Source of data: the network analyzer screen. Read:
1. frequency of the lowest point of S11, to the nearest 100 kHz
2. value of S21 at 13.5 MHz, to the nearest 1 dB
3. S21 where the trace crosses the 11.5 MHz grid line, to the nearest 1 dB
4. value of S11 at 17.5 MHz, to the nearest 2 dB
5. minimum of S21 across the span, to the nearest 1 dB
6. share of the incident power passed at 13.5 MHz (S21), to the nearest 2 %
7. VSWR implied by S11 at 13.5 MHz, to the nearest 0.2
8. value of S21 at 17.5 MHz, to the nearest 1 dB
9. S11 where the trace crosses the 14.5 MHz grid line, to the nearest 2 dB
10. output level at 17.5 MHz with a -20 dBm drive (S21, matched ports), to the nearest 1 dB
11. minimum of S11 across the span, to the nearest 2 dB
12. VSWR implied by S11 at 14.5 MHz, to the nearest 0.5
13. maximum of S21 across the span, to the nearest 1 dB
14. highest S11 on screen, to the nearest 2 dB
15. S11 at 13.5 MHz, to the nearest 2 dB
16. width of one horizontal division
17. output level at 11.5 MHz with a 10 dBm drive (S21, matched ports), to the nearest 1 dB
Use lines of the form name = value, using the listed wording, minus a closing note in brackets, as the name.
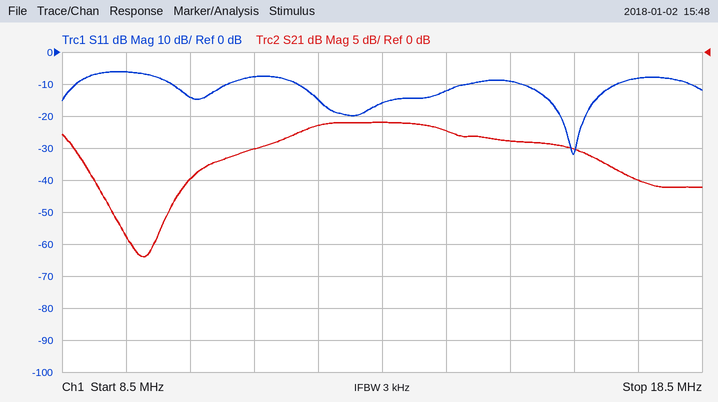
frequency of the lowest point of S11, to the nearest 100 kHz = 16.5 MHz
value of S21 at 13.5 MHz, to the nearest 1 dB = -11 dB
S21 where the trace crosses the 11.5 MHz grid line, to the nearest 1 dB = -15 dB
value of S11 at 17.5 MHz, to the nearest 2 dB = -8 dB
minimum of S21 across the span, to the nearest 1 dB = -32 dB
share of the incident power passed at 13.5 MHz (S21), to the nearest 2 % = 8 %
VSWR implied by S11 at 13.5 MHz, to the nearest 0.2 = 1.4
value of S21 at 17.5 MHz, to the nearest 1 dB = -20 dB
S11 where the trace crosses the 14.5 MHz grid line, to the nearest 2 dB = -12 dB
output level at 17.5 MHz with a -20 dBm drive (S21, matched ports), to the nearest 1 dB = -40 dBm
minimum of S11 across the span, to the nearest 2 dB = -32 dB
VSWR implied by S11 at 14.5 MHz, to the nearest 0.5 = 1.5
maximum of S21 across the span, to the nearest 1 dB = -11 dB
highest S11 on screen, to the nearest 2 dB = -6 dB
S11 at 13.5 MHz, to the nearest 2 dB = -16 dB
width of one horizontal division = 1 MHz
output level at 11.5 MHz with a 10 dBm drive (S21, matched ports), to the nearest 1 dB = -5 dBm
